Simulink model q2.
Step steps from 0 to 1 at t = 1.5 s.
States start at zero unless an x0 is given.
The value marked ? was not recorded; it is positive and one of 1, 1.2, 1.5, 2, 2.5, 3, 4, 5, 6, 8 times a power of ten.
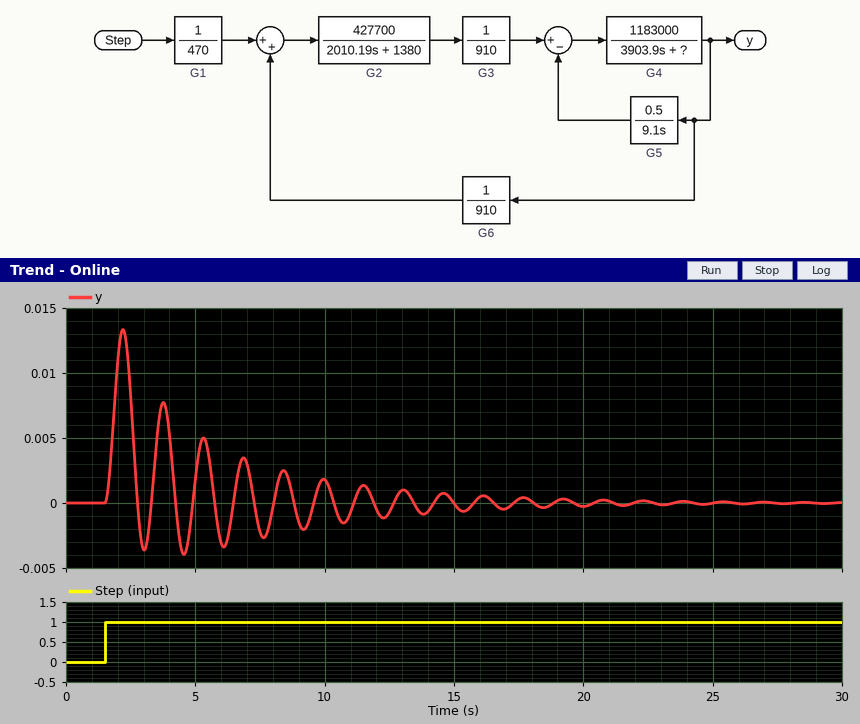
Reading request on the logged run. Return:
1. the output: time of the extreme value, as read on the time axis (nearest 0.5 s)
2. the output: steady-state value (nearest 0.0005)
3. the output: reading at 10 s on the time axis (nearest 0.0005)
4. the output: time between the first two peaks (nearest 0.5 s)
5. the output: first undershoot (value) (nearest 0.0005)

2.0 s
0.0000
0.0020
1.5 s
-0.0035
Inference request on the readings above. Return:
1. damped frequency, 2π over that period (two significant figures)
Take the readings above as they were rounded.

4.2 rad/s
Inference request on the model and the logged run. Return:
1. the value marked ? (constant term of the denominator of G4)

1500
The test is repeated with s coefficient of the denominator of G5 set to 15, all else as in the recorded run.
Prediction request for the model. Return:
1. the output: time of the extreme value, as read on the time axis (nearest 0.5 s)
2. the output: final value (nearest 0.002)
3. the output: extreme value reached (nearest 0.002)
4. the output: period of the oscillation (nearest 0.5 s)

2.5 s
0.000
0.020
2.0 s
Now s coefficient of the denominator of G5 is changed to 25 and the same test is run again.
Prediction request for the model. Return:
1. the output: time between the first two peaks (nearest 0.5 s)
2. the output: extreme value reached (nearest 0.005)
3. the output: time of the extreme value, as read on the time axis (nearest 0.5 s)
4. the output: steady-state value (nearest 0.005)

2.5 s
0.030
2.5 s
0.000
